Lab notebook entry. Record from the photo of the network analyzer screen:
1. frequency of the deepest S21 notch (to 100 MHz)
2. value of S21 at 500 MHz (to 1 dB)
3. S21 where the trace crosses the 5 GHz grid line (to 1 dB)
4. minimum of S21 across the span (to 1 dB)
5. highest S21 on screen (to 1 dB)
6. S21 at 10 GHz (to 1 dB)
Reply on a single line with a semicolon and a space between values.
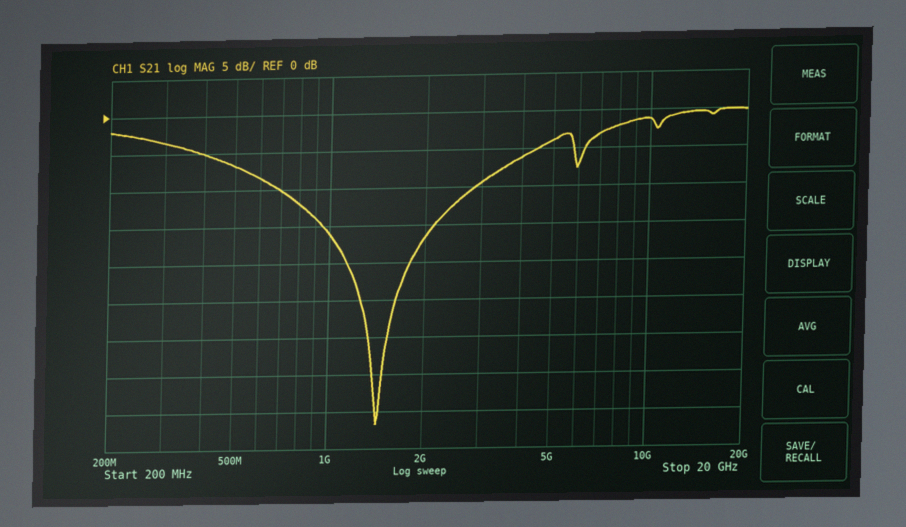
1.4 GHz; -7 dB; -4 dB; -42 dB; 0 dB; -1 dB
